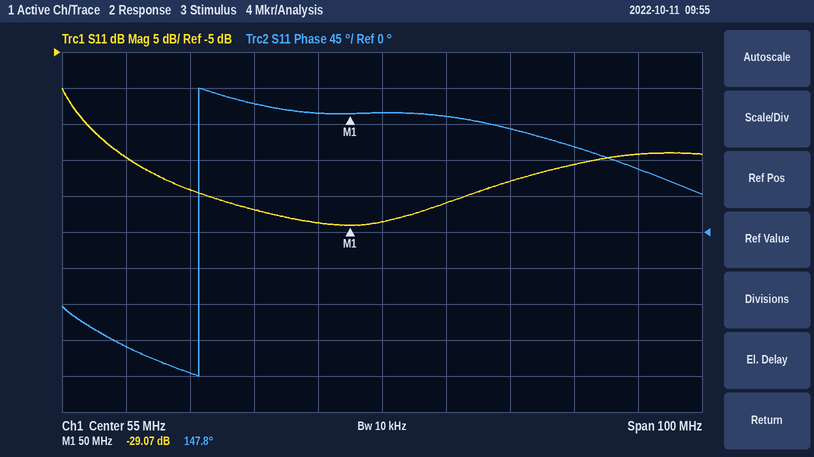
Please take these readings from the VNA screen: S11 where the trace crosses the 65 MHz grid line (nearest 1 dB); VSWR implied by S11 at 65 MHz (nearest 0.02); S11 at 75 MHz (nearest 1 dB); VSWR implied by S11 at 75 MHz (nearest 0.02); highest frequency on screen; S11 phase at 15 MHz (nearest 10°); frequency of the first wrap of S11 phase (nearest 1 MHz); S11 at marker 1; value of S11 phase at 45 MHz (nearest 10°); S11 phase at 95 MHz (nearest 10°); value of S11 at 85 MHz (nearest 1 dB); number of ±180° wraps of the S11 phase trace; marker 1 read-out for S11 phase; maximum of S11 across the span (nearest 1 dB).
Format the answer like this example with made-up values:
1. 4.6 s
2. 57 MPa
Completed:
1. -26 dB
2. 1.10
3. -23 dB
4. 1.16
5. 105 MHz
6. -140°
7. 26 MHz
8. -29.07 dB
9. 150°
10. 80°
11. -21 dB
12. 1
13. 147.8°
14. -10 dB
